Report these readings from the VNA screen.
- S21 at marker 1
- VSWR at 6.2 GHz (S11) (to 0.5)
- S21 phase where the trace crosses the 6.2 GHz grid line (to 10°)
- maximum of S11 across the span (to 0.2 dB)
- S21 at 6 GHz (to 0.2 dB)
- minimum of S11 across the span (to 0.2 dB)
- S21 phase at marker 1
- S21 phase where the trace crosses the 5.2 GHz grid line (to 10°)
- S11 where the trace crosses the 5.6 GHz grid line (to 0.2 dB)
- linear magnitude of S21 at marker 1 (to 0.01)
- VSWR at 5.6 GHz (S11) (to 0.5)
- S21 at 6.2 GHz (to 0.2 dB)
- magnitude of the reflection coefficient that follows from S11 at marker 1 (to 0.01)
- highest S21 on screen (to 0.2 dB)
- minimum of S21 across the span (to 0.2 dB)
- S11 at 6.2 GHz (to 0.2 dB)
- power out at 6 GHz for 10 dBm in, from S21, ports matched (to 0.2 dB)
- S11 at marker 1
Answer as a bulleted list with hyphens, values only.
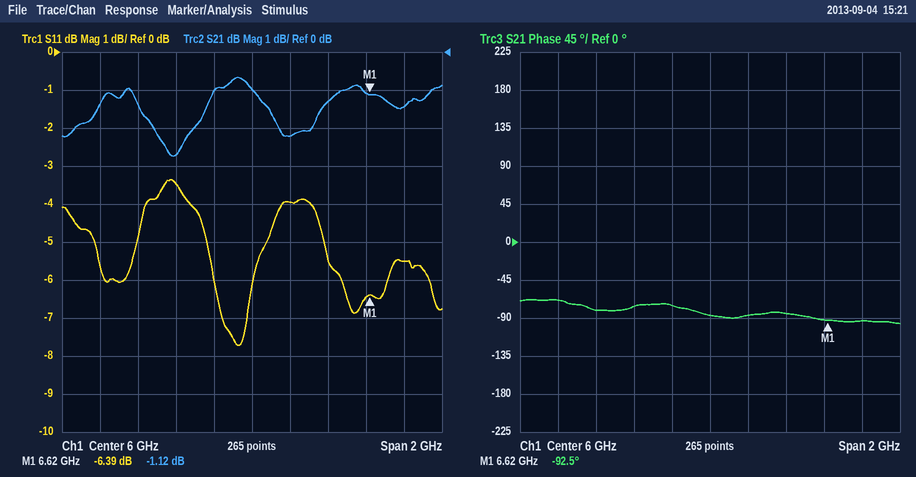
- -1.12 dB
- 4.5
- -90°
- -3.4 dB
- -1.0 dB
- -7.8 dB
- -92.5°
- -70°
- -3.4 dB
- 0.88
- 5.0
- -2.2 dB
- 0.48
- -0.6 dB
- -2.8 dB
- -4.0 dB
- 9.0 dBm
- -6.39 dB
